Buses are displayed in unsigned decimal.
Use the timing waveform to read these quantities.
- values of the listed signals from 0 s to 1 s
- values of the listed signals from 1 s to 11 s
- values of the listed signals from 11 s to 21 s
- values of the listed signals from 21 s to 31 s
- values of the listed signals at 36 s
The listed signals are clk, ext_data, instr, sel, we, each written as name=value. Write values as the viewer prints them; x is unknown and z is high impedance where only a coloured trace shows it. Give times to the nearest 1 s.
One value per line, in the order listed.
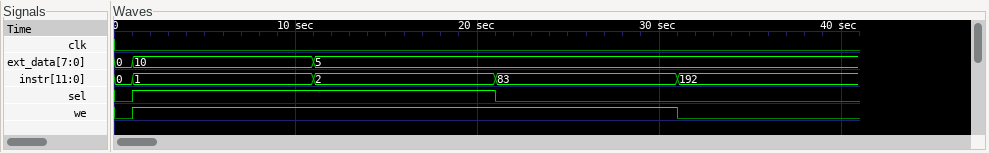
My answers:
clk=0, ext_data=0, instr=0, sel=0, we=0
clk=0, ext_data=10, instr=1, sel=1, we=1
clk=0, ext_data=5, instr=2, sel=1, we=1
clk=0, ext_data=5, instr=83, sel=0, we=1
clk=0, ext_data=5, instr=192, sel=0, we=0
